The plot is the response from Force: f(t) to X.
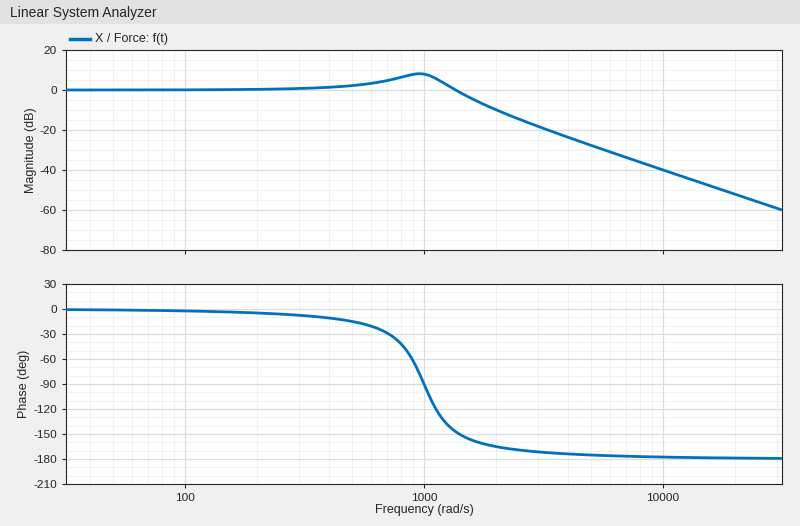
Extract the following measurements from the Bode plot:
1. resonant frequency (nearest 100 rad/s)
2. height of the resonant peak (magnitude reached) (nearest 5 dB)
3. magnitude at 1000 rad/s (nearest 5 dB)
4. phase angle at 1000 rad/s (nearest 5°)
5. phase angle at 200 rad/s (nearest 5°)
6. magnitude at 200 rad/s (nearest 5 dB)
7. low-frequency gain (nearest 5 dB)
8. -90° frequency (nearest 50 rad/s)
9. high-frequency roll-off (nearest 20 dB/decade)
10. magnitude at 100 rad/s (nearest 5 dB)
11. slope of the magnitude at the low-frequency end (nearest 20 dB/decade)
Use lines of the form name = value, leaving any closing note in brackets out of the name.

resonant frequency = 1000 rad/s
height of the resonant peak (magnitude reached) = 10 dB
magnitude at 1000 rad/s = 10 dB
phase angle at 1000 rad/s = -90°
phase angle at 200 rad/s = -5°
magnitude at 200 rad/s = 0 dB
low-frequency gain = 0 dB
-90° frequency = 1000 rad/s
high-frequency roll-off = -40 dB/decade
magnitude at 100 rad/s = 0 dB
slope of the magnitude at the low-frequency end = 0 dB/decade
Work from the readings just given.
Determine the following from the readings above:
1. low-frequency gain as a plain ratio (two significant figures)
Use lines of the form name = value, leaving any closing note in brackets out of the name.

low-frequency gain as a plain ratio = 1.0
